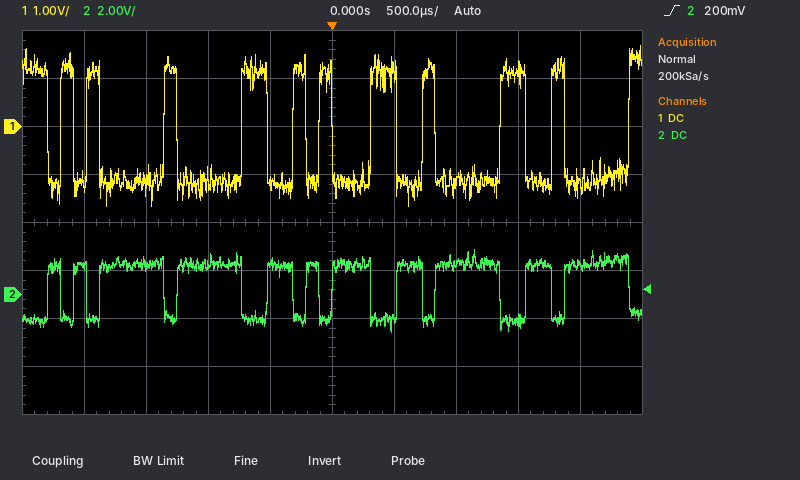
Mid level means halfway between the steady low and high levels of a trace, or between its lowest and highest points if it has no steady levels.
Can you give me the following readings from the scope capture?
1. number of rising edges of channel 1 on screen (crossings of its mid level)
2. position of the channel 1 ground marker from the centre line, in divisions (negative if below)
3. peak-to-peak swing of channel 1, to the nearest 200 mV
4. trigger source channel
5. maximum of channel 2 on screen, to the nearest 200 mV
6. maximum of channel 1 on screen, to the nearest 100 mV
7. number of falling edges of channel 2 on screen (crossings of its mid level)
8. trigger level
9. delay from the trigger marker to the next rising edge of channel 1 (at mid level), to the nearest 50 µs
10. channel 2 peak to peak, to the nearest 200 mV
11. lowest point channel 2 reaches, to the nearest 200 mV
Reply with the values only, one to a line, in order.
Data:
11
+2.0 div
3.4 V
channel 2
1.8 V
1.7 V
11
200 mV
300 µs
3.4 V
-1.6 V
